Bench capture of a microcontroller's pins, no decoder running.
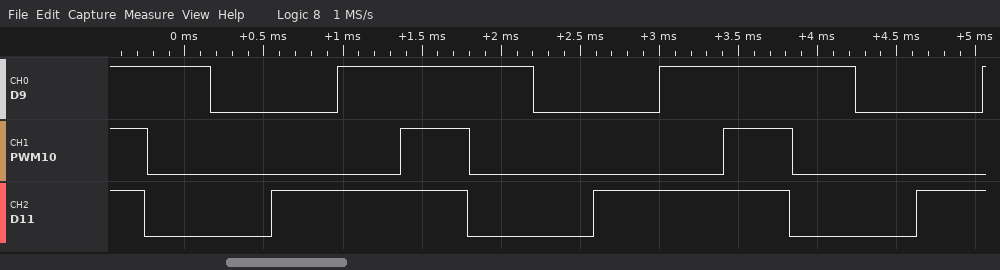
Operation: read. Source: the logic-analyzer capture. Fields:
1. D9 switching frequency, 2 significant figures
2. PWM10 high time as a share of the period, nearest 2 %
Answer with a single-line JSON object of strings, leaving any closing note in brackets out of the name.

{"D9 switching frequency, 2 significant figures": "490 Hz", "PWM10 high time as a share of the period, nearest 2 %": "22 %"}
